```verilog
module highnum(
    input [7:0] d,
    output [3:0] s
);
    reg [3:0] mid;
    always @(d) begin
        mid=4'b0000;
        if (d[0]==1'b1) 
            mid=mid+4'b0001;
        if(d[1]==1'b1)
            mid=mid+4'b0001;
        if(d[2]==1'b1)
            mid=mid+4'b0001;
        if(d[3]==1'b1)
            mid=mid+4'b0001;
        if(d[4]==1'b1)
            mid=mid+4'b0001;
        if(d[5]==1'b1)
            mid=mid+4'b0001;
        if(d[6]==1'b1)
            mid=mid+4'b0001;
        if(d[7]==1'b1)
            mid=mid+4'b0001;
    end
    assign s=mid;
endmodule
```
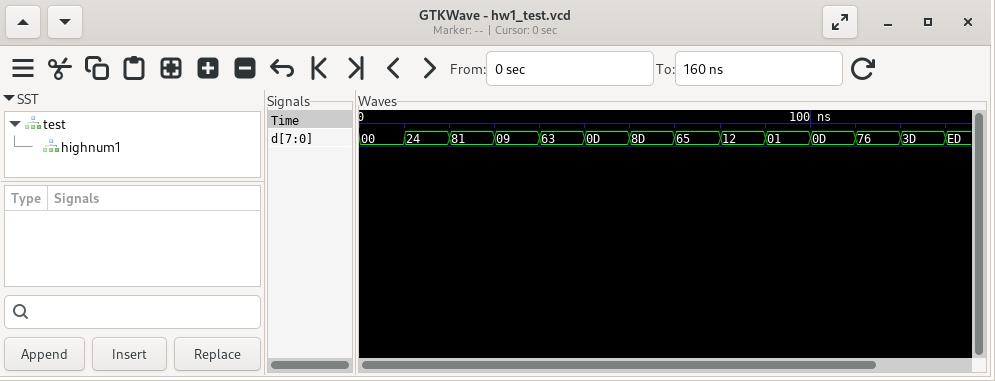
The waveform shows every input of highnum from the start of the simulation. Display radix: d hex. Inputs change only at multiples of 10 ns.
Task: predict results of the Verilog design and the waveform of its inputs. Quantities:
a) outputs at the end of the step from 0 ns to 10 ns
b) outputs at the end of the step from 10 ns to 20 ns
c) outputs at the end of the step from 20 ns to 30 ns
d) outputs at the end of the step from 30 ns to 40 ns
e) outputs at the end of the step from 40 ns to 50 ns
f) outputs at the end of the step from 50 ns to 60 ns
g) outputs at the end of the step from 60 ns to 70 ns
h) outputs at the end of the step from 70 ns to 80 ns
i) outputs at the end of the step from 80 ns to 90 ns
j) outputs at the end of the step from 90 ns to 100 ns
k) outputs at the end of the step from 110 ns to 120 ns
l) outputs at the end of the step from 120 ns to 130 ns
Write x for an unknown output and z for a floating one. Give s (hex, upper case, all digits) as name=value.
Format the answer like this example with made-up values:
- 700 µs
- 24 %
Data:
- s=0
- s=2
- s=2
- s=2
- s=4
- s=3
- s=4
- s=4
- s=2
- s=1
- s=5
- s=5
